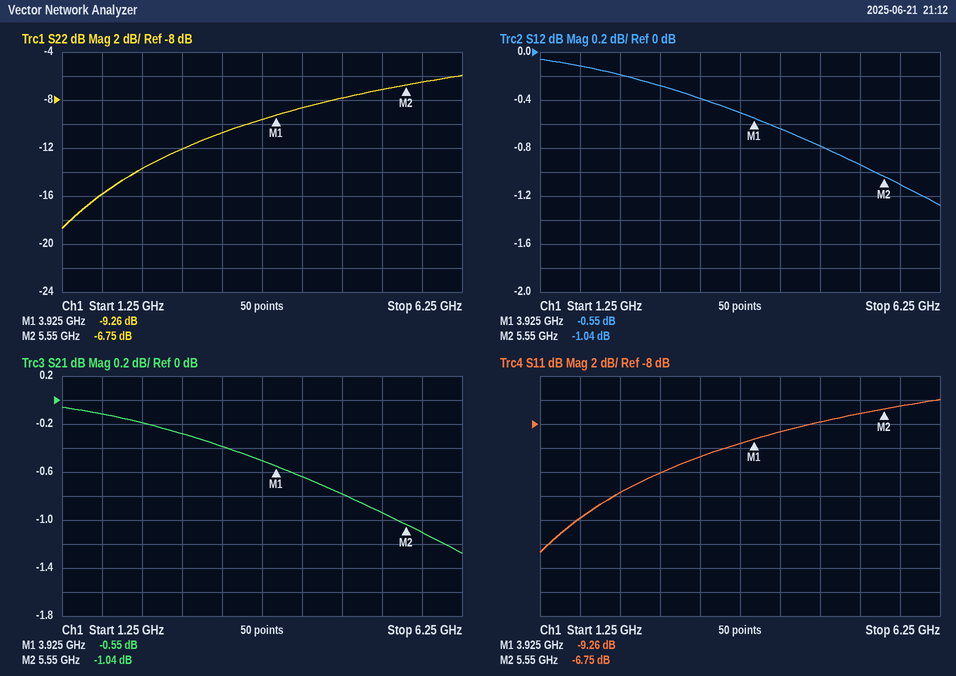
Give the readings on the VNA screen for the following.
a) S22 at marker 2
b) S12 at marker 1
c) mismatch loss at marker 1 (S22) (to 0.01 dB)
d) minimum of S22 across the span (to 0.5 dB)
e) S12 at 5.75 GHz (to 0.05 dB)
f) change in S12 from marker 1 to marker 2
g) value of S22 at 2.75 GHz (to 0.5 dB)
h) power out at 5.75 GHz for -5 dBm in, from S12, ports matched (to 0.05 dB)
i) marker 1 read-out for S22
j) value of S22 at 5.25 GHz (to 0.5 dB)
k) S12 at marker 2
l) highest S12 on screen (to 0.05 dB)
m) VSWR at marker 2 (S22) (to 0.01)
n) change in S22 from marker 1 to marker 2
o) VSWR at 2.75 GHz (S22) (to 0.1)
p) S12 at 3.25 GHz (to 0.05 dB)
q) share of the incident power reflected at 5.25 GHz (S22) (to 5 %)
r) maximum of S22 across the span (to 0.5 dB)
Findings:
-6.75 dB
-0.55 dB
0.55 dB
-18.5 dB
-1.10 dB
-0.49 dB
-12.0 dB
-6.10 dBm
-9.26 dB
-7.0 dB
-1.04 dB
-0.05 dB
2.70
2.51 dB
1.7
-0.40 dB
20 %
-6.0 dB
